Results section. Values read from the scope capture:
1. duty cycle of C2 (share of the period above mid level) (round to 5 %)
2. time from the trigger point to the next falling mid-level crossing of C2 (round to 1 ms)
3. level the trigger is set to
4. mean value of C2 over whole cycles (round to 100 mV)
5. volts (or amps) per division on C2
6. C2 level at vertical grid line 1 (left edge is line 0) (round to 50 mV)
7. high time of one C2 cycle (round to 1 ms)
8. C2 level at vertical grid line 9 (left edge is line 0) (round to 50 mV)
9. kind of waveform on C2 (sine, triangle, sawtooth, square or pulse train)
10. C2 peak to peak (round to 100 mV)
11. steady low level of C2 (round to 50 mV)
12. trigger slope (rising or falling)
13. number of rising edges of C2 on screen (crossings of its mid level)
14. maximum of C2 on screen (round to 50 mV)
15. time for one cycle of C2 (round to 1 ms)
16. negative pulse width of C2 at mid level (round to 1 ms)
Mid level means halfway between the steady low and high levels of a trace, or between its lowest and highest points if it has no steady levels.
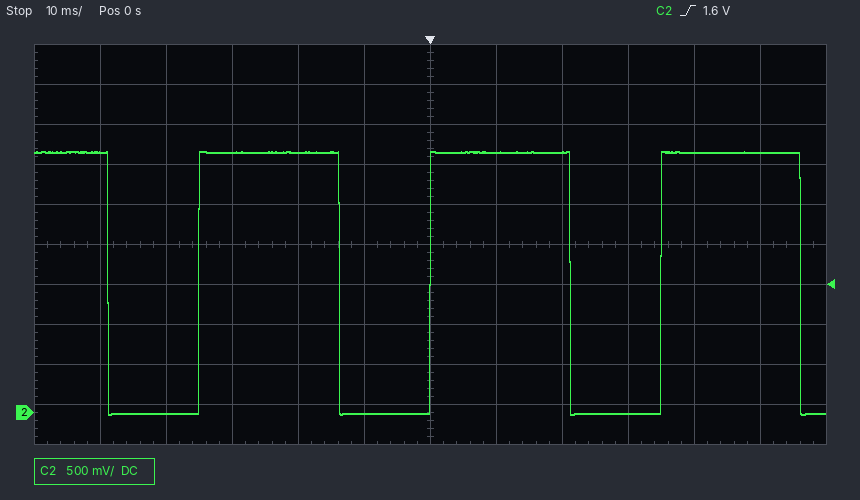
60 %
21 ms
1.6 V
2.0 V
500 mV
3.25 V
21 ms
0 mV
pulse train
3.30 V
0 mV
rising
3
3.25 V
35 ms
14 ms
